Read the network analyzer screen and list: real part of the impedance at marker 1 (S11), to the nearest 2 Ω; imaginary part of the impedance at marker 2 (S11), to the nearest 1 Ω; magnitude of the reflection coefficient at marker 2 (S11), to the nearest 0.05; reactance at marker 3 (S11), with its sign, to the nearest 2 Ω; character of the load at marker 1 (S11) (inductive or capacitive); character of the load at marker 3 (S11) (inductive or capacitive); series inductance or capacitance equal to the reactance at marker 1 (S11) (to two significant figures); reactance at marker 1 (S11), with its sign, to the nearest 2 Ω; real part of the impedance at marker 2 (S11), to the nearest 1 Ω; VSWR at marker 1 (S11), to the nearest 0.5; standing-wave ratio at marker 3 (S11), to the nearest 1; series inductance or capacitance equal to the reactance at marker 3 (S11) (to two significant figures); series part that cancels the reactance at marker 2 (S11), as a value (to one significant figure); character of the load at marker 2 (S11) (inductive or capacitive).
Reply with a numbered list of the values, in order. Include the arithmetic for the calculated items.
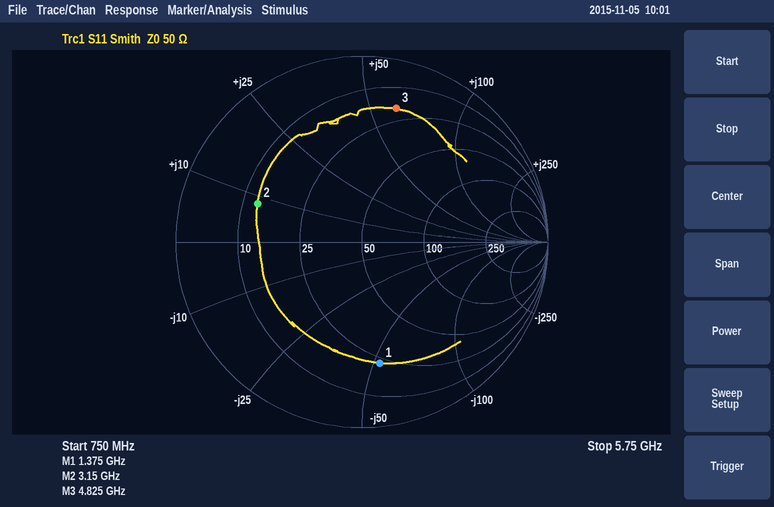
1. 22 Ω
2. +8 Ω
3. 0.60
4. +60 Ω
5. capacitive
6. inductive
7. C = 1/(2π × 1.375 GHz × 52 Ω) ≈ 2.2 pF
8. -52 Ω
9. 13 Ω
10. 5.0
11. 7
12. L = 60 Ω/(2π × 4.825 GHz) ≈ 2.0 nH
13. C = 1/(2π × 3.15 GHz × 8 Ω) ≈ 6 pF
14. inductive
